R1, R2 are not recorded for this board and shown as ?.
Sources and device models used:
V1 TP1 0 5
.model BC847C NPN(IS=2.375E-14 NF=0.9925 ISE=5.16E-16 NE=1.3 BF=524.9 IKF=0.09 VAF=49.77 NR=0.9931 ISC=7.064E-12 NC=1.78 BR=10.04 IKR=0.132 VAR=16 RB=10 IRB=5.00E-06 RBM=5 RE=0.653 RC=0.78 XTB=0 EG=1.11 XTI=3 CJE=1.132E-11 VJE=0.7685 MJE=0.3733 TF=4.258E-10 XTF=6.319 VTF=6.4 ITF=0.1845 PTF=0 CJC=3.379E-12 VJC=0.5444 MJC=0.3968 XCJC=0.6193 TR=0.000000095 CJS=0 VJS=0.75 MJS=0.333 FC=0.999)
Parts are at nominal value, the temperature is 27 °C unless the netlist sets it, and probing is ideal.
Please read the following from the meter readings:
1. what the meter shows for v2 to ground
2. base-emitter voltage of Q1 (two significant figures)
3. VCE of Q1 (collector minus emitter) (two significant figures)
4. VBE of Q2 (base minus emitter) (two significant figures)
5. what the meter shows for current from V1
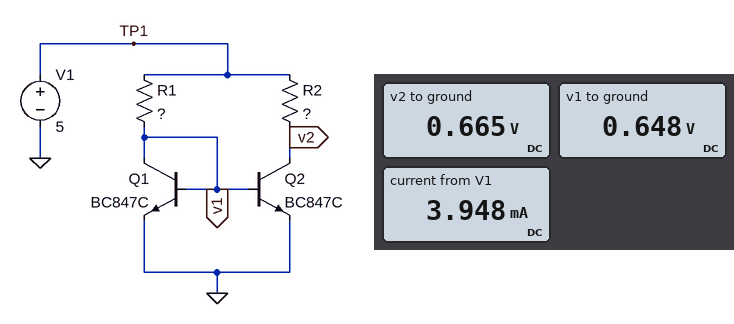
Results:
0.665 V
650 mV
650 mV
650 mV
3.948 mA
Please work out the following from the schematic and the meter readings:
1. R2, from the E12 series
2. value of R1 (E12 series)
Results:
2.2 kΩ
2.2 kΩ
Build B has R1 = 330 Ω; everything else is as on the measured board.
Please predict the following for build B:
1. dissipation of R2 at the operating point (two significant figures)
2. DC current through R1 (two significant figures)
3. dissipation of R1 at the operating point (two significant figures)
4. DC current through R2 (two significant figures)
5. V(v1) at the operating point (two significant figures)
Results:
11 mW
13 mA
56 mW
2.3 mA
700 mV
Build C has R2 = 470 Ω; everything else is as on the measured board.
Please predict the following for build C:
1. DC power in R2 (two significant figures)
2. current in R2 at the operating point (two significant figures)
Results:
2.1 mW
2.1 mA
